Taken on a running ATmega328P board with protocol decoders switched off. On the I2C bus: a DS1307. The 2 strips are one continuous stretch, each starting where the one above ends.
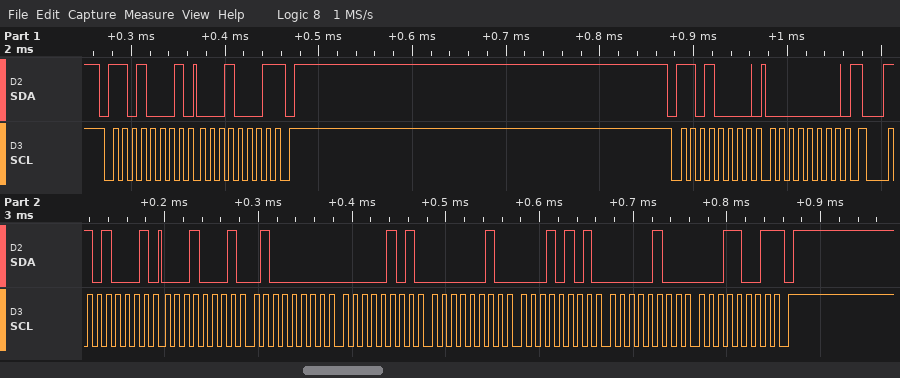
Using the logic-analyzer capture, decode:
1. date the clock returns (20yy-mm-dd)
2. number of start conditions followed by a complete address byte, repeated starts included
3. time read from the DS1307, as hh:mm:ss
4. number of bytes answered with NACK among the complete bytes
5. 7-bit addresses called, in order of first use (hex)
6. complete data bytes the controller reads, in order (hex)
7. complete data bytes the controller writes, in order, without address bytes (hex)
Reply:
2019-04-15
3
05:40:11
2
0x68
11 11 40 05 02 15 04 19
00
